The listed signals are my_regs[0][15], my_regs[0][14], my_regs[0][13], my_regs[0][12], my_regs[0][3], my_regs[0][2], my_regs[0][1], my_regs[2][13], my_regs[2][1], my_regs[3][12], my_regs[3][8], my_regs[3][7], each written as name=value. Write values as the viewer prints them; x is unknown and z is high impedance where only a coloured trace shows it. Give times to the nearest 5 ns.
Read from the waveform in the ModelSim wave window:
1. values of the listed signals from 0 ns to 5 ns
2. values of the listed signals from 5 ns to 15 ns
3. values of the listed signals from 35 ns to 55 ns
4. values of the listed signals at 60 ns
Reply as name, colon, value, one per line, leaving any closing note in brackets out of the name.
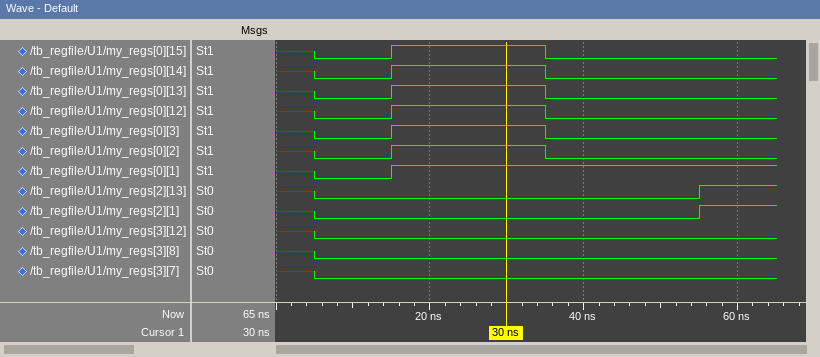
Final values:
values of the listed signals from 0 ns to 5 ns: my_regs[0][15]=x, my_regs[0][14]=x, my_regs[0][13]=x, my_regs[0][12]=x, my_regs[0][3]=x, my_regs[0][2]=x, my_regs[0][1]=x, my_regs[2][13]=x, my_regs[2][1]=x, my_regs[3][12]=x, my_regs[3][8]=x, my_regs[3][7]=x
values of the listed signals from 5 ns to 15 ns: my_regs[0][15]=0, my_regs[0][14]=0, my_regs[0][13]=0, my_regs[0][12]=0, my_regs[0][3]=0, my_regs[0][2]=0, my_regs[0][1]=0, my_regs[2][13]=0, my_regs[2][1]=0, my_regs[3][12]=0, my_regs[3][8]=0, my_regs[3][7]=0
values of the listed signals from 35 ns to 55 ns: my_regs[0][15]=0, my_regs[0][14]=0, my_regs[0][13]=0, my_regs[0][12]=0, my_regs[0][3]=0, my_regs[0][2]=0, my_regs[0][1]=1, my_regs[2][13]=0, my_regs[2][1]=0, my_regs[3][12]=0, my_regs[3][8]=0, my_regs[3][7]=0
values of the listed signals at 60 ns: my_regs[0][15]=0, my_regs[0][14]=0, my_regs[0][13]=0, my_regs[0][12]=0, my_regs[0][3]=0, my_regs[0][2]=0, my_regs[0][1]=1, my_regs[2][13]=1, my_regs[2][1]=1, my_regs[3][12]=0, my_regs[3][8]=0, my_regs[3][7]=0
